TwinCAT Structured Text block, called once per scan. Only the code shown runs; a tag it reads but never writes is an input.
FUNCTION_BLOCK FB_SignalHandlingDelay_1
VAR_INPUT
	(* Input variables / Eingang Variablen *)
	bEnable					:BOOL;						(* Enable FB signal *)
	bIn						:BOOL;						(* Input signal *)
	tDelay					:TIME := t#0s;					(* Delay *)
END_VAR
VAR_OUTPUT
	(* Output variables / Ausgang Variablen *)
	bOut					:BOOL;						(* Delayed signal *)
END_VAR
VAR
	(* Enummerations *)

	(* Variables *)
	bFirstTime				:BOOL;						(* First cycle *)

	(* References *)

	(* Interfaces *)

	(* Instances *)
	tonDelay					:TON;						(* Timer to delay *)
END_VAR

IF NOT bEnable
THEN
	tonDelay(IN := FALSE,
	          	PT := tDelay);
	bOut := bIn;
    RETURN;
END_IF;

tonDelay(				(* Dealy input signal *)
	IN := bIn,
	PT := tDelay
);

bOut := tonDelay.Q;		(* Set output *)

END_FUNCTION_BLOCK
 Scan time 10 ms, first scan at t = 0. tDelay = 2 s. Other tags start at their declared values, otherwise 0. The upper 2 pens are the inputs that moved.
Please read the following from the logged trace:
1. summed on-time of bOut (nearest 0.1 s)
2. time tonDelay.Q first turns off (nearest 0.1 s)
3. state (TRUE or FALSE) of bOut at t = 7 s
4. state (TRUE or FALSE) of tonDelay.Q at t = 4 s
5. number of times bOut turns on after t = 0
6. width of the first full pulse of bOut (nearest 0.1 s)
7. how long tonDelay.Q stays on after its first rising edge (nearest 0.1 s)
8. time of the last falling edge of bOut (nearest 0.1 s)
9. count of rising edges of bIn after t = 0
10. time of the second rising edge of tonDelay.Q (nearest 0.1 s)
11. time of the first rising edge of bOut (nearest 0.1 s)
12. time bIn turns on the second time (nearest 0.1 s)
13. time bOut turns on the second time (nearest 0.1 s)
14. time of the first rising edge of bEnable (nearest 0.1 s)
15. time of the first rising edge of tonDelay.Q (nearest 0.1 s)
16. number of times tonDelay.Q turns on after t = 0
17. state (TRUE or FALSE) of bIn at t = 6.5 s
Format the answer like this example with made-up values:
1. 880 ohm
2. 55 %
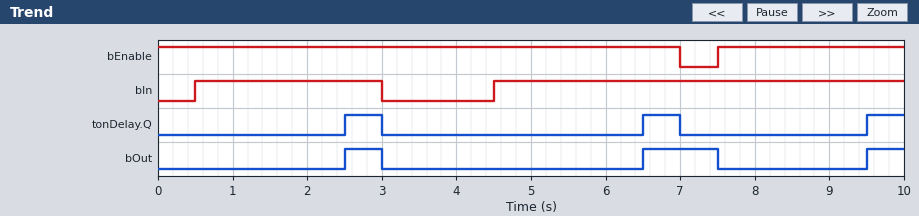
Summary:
1. 2.0 s
2. 3.0 s
3. TRUE
4. FALSE
5. 3
6. 0.5 s
7. 0.5 s
8. 7.5 s
9. 2
10. 6.5 s
11. 2.5 s
12. 4.5 s
13. 6.5 s
14. 7.5 s
15. 2.5 s
16. 3
17. TRUE
